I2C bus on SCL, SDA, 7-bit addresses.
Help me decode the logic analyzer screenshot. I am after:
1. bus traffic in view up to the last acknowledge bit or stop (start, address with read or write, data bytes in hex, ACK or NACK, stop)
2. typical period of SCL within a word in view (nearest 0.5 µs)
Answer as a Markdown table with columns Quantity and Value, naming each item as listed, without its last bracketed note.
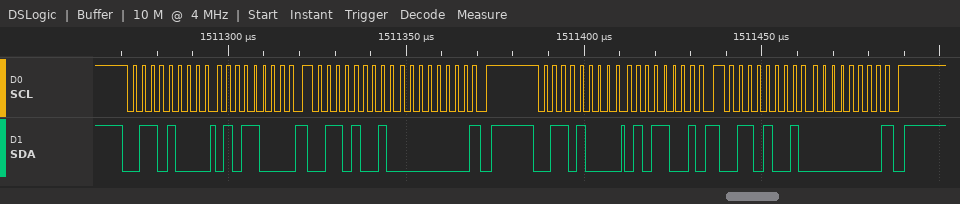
| Quantity | Value |
|---|---|
| bus traffic in view up to the last acknowledge bit or stop | start, address 34 write ACK, 58 ACK, repeated start, address 34 read ACK, 00 NACK, stop, start, address 34 write ACK, 59 ACK, repeated start, address 34 read ACK, 00 NACK, stop |
| typical period of SCL within a word in view | 2.5 µs |
